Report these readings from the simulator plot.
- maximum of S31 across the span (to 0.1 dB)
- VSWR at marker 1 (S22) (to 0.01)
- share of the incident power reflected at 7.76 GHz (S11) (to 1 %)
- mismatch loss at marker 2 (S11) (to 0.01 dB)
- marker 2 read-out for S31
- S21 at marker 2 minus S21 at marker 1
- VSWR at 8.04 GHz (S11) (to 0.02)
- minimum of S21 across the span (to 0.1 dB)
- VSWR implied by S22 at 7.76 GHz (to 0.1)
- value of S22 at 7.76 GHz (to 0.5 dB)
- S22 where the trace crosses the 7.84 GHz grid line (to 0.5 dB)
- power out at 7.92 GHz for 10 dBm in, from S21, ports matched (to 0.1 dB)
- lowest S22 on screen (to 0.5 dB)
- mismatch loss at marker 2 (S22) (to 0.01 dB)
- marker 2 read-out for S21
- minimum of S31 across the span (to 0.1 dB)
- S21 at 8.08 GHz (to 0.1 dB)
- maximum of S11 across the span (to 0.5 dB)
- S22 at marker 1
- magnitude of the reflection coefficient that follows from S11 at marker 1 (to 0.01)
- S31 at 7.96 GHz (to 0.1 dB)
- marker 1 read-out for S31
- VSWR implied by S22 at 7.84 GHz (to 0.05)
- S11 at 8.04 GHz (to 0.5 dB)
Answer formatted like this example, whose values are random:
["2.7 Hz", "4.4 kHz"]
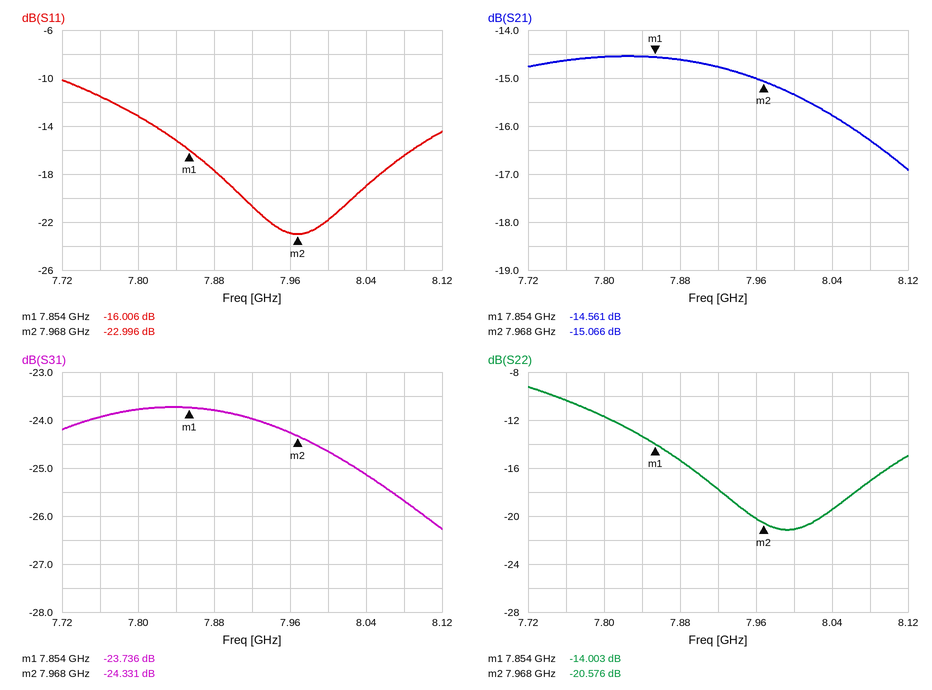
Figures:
["-23.7 dB", "1.50", "7 %", "0.02 dB", "-24.331 dB", "-0.505 dB", "1.26", "-16.9 dB", "1.9", "-10.5 dB", "-13.5 dB", "-4.8 dBm", "-21.0 dB", "0.04 dB", "-15.066 dB", "-26.3 dB", "-16.3 dB", "-10.0 dB", "-14.003 dB", "0.16", "-24.3 dB", "-23.736 dB", "1.55", "-19.0 dB"]
